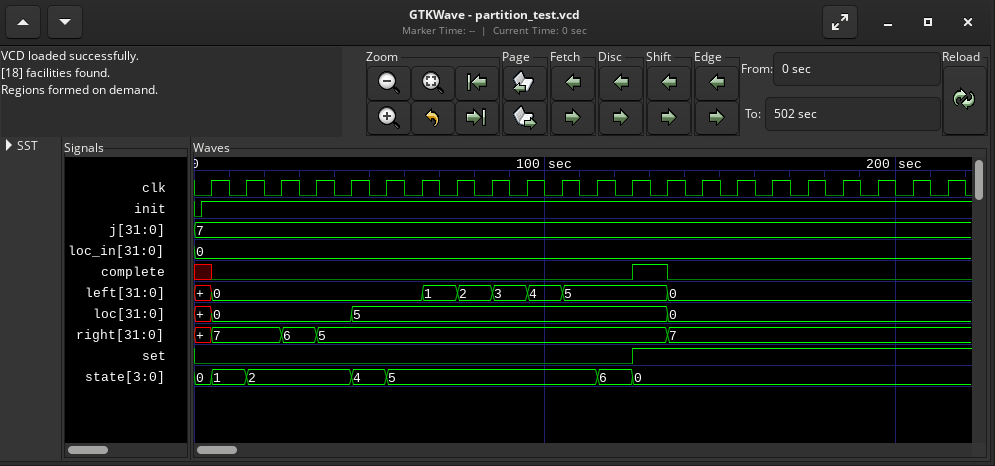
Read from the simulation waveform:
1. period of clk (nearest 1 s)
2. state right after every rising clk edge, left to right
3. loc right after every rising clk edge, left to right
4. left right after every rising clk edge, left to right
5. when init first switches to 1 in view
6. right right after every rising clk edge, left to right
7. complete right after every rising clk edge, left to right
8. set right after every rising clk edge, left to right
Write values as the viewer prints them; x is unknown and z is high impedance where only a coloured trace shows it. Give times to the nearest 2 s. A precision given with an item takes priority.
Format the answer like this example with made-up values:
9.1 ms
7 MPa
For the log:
10 s
1, 2, 2, 2, 4, 5, 5, 5, 5, 5, 5, 6, 0, 0, 0, 0, 0, 0, 0, 0, 0, 0
0, 0, 0, 0, 5, 5, 5, 5, 5, 5, 5, 5, 5, 0, 0, 0, 0, 0, 0, 0, 0, 0
0, 0, 0, 0, 0, 0, 1, 2, 3, 4, 5, 5, 5, 0, 0, 0, 0, 0, 0, 0, 0, 0
2 s
7, 7, 6, 5, 5, 5, 5, 5, 5, 5, 5, 5, 5, 7, 7, 7, 7, 7, 7, 7, 7, 7
0 0 0 0 0 0 0 0 0 0 0 0 1 0 0 0 0 0 0 0 0 0
0 0 0 0 0 0 0 0 0 0 0 0 1 1 1 1 1 1 1 1 1 1
